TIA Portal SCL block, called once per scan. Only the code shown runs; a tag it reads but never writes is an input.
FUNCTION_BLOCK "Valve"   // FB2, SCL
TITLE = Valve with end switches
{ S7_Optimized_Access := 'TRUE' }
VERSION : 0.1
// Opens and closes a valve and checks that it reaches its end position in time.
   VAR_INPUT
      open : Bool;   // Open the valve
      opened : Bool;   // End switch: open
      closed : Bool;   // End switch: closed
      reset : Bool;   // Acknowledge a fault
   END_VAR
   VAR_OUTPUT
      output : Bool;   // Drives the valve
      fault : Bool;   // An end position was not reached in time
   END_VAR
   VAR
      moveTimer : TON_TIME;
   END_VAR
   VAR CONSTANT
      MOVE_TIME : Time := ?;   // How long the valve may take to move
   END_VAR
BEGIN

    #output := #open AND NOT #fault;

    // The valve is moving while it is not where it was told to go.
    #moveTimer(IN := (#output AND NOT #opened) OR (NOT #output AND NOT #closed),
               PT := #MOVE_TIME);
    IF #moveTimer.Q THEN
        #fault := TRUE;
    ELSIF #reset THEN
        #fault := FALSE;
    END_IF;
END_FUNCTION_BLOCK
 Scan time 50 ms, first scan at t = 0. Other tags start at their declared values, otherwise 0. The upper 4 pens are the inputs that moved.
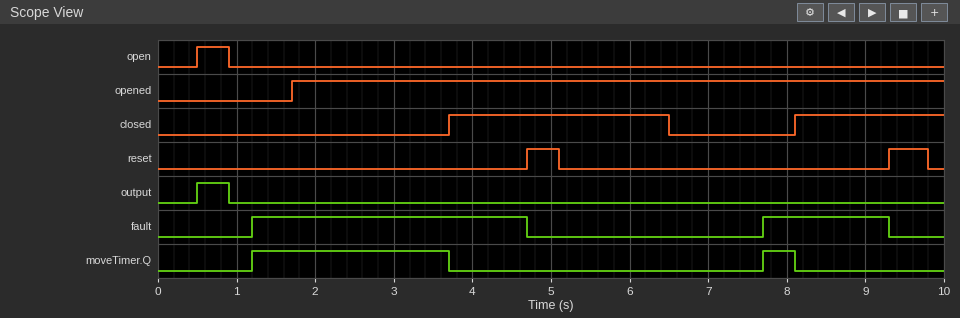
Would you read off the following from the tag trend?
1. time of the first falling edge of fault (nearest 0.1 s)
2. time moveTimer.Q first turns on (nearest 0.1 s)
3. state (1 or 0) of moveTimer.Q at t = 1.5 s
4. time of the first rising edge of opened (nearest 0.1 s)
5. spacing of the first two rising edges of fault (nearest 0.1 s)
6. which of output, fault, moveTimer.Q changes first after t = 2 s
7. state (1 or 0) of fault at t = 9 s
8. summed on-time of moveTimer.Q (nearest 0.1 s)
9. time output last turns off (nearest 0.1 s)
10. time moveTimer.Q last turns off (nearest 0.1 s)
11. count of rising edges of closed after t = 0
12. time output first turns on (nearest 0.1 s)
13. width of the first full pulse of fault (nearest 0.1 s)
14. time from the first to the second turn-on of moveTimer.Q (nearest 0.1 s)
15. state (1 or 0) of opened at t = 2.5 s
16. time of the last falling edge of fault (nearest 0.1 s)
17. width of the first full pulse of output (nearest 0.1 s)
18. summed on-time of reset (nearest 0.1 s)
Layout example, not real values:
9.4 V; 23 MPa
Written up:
4.7 s; 1.2 s; 1; 1.7 s; 6.5 s; moveTimer.Q; 1; 2.9 s; 0.9 s; 8.1 s; 2; 0.5 s; 3.5 s; 6.5 s; 1; 9.3 s; 0.4 s; 0.9 s
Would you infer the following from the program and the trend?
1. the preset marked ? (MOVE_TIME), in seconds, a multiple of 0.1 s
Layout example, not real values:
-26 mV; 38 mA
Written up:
1.2 s
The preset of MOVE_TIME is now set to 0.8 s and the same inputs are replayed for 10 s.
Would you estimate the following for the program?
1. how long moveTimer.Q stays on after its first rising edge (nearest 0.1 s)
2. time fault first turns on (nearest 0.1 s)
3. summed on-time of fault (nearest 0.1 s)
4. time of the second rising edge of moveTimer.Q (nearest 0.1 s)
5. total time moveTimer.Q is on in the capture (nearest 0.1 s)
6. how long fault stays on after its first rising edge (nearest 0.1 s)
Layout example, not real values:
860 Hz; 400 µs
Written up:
2.9 s; 0.8 s; 5.9 s; 7.3 s; 3.7 s; 3.9 s
